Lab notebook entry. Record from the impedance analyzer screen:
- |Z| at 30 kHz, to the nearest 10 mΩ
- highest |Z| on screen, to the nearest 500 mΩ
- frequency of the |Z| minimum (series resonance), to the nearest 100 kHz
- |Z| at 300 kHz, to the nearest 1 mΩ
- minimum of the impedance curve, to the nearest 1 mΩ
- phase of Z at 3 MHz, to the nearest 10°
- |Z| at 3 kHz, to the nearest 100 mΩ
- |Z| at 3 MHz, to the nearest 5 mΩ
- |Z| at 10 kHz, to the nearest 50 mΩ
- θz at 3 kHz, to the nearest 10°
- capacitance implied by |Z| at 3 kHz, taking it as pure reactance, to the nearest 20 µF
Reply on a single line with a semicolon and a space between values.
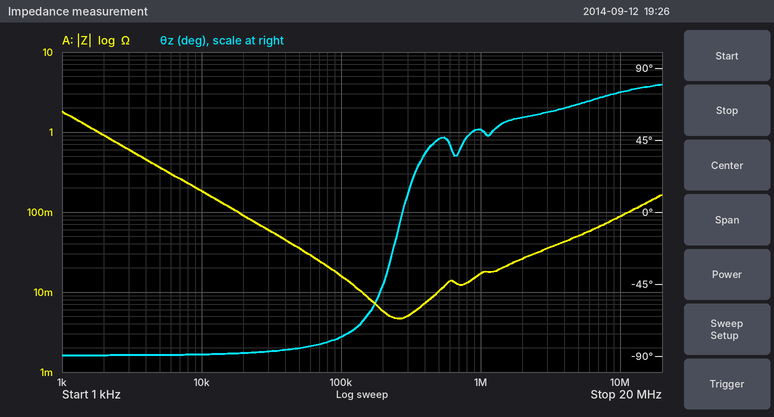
60 mΩ; 2.0 Ω; 300 kHz; 5 mΩ; 5 mΩ; 60°; 600 mΩ; 35 mΩ; 200 mΩ; -90°; 80 µF
